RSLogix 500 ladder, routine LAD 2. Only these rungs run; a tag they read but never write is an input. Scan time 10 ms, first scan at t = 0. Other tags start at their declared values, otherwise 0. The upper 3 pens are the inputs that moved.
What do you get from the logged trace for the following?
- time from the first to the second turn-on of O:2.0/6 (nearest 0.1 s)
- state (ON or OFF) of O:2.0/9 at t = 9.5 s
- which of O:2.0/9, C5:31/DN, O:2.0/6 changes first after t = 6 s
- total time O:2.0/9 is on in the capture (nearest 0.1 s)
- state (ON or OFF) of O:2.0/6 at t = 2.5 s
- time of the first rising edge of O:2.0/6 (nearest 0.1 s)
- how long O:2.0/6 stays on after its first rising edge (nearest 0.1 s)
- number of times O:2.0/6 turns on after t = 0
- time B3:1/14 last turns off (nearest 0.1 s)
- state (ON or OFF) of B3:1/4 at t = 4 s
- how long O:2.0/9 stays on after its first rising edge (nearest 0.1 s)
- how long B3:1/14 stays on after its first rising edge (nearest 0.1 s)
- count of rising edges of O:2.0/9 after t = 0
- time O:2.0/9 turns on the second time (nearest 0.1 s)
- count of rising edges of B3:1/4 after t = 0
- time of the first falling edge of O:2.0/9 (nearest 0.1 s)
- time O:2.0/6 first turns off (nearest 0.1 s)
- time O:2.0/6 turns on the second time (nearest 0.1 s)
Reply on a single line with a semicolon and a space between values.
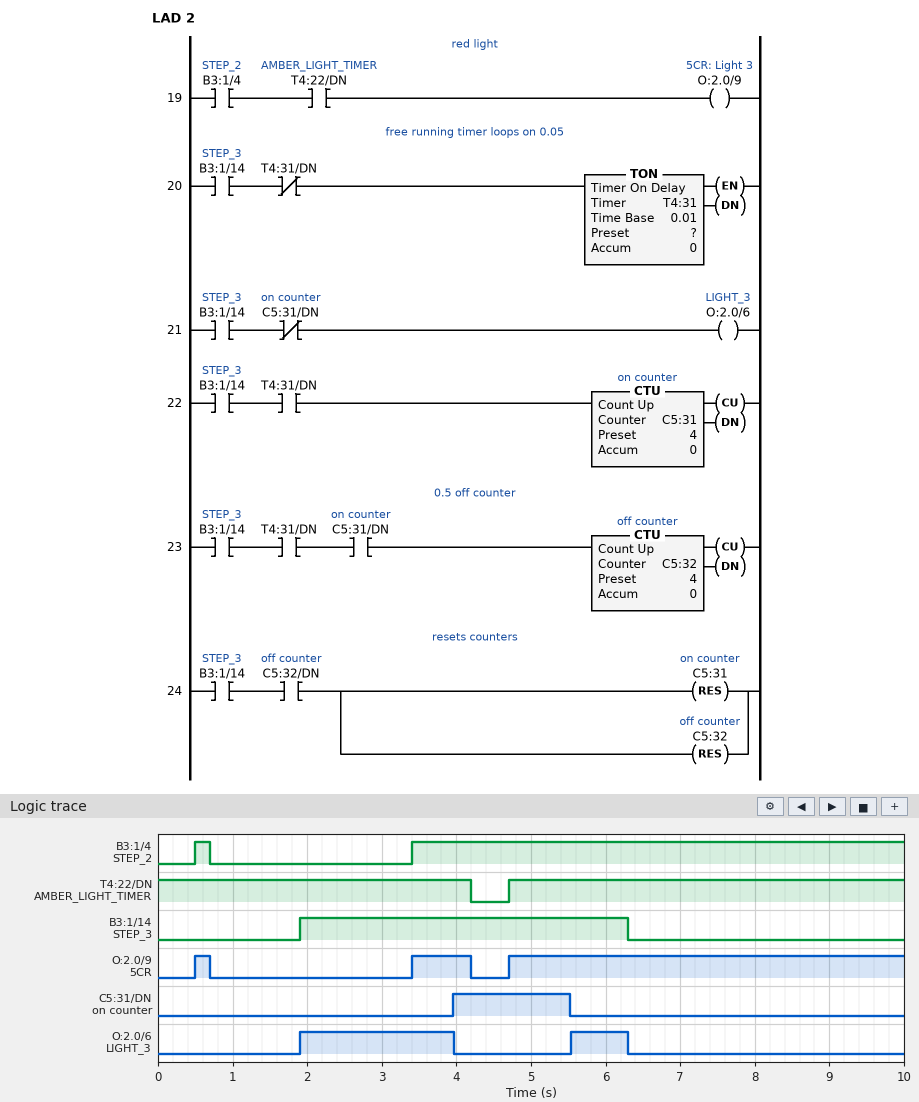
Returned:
3.6 s; ON; O:2.0/6; 6.3 s; ON; 1.9 s; 2.1 s; 2; 6.3 s; ON; 0.2 s; 4.4 s; 3; 3.4 s; 2; 0.7 s; 4.0 s; 5.5 s
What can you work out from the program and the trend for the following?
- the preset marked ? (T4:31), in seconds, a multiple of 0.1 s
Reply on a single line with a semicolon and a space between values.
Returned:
0.5 s
